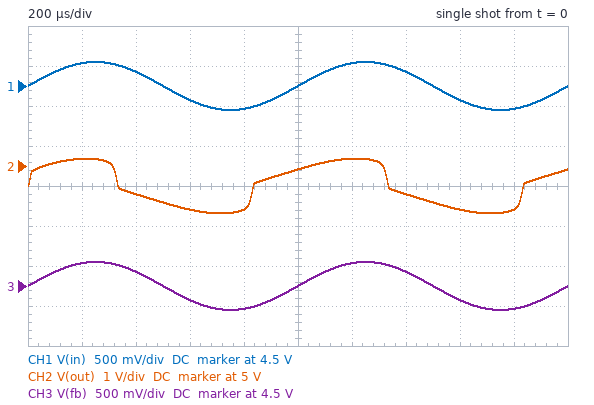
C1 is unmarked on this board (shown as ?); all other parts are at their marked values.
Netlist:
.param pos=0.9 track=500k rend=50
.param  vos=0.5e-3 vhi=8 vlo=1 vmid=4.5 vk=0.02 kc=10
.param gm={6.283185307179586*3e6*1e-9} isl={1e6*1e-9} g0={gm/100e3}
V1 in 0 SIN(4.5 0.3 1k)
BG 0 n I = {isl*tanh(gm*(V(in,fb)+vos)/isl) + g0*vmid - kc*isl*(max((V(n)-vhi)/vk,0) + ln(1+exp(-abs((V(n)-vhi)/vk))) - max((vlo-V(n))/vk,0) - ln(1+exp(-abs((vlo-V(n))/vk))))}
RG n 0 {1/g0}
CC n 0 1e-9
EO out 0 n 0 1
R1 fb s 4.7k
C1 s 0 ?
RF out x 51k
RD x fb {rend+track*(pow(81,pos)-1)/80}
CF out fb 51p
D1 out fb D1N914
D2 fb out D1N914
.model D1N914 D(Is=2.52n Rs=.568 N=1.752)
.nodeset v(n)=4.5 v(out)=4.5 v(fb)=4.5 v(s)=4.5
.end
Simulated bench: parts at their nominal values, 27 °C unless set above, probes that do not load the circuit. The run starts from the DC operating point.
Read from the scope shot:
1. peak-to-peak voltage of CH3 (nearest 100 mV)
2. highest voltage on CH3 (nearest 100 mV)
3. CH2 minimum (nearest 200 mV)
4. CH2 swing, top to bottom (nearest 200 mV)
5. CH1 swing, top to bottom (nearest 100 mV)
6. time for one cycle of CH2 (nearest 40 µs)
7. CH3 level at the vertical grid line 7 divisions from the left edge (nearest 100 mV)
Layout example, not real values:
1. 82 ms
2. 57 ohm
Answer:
1. 600 mV
2. 4.8 V
3. 3.8 V
4. 1.4 V
5. 600 mV
6. 1.00 ms
7. 4.7 V
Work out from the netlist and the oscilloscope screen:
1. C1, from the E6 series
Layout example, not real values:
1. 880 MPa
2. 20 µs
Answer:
1. 15 nF
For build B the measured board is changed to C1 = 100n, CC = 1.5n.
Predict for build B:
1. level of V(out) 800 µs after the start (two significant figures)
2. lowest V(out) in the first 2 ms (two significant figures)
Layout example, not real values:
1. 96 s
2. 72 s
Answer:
1. 3.8 V
2. 3.7 V
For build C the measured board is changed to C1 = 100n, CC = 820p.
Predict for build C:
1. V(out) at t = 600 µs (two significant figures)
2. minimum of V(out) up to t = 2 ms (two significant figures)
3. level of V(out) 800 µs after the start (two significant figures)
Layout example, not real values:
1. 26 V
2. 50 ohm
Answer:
1. 3.9 V
2. 3.7 V
3. 3.8 V
